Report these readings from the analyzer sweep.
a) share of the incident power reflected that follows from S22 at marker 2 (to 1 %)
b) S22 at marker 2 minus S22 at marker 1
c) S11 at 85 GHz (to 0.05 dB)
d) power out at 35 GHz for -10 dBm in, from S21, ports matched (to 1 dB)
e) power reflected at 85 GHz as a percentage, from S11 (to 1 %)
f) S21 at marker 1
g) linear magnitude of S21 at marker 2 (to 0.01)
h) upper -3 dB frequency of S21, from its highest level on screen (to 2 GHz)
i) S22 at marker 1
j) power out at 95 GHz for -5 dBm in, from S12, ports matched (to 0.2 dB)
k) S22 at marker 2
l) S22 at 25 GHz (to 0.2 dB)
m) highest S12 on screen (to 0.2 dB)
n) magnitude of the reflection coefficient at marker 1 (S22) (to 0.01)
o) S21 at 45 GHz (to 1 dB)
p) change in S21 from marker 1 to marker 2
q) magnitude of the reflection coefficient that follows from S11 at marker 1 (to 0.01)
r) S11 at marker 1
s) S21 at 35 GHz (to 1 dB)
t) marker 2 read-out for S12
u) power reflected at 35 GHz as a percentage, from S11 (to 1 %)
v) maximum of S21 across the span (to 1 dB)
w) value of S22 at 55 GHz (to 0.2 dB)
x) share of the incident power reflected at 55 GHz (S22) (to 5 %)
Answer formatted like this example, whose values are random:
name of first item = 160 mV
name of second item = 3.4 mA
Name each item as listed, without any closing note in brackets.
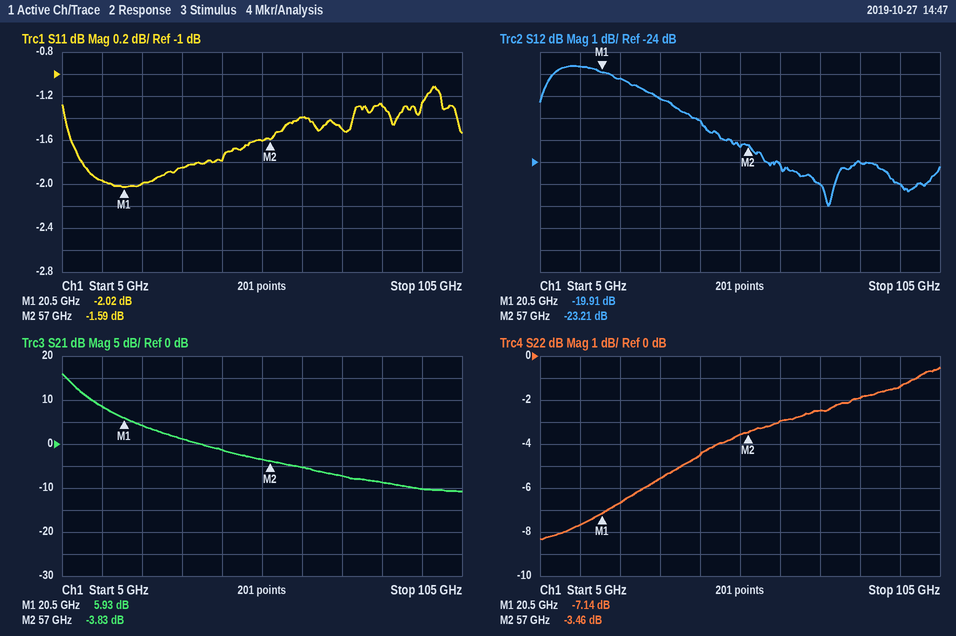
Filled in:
share of the incident power reflected that follows from S22 at marker 2 = 45 %
S22 at marker 2 minus S22 at marker 1 = 3.68 dB
S11 at 85 GHz = -1.30 dB
power out at 35 GHz for -10 dBm in, from S21, ports matched = -9 dBm
power reflected at 85 GHz as a percentage, from S11 = 74 %
S21 at marker 1 = 5.93 dB
linear magnitude of S21 at marker 2 = 0.64
upper -3 dB frequency of S21, from its highest level on screen = 8 GHz
S22 at marker 1 = -7.14 dB
power out at 95 GHz for -5 dBm in, from S12, ports matched = -30.0 dBm
S22 at marker 2 = -3.46 dB
S22 at 25 GHz = -6.6 dB
highest S12 on screen = -19.6 dB
magnitude of the reflection coefficient at marker 1 (S22) = 0.44
S21 at 45 GHz = -1 dB
change in S21 from marker 1 to marker 2 = -9.76 dB
magnitude of the reflection coefficient that follows from S11 at marker 1 = 0.79
S11 at marker 1 = -2.02 dB
S21 at 35 GHz = 1 dB
marker 2 read-out for S12 = -23.21 dB
power reflected at 35 GHz as a percentage, from S11 = 65 %
maximum of S21 across the span = 16 dB
value of S22 at 55 GHz = -3.6 dB
share of the incident power reflected at 55 GHz (S22) = 45 %
